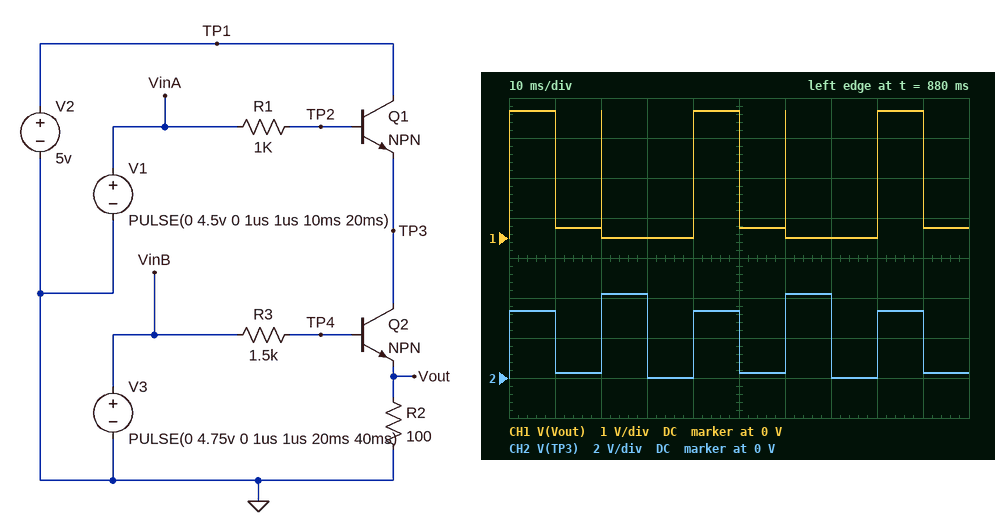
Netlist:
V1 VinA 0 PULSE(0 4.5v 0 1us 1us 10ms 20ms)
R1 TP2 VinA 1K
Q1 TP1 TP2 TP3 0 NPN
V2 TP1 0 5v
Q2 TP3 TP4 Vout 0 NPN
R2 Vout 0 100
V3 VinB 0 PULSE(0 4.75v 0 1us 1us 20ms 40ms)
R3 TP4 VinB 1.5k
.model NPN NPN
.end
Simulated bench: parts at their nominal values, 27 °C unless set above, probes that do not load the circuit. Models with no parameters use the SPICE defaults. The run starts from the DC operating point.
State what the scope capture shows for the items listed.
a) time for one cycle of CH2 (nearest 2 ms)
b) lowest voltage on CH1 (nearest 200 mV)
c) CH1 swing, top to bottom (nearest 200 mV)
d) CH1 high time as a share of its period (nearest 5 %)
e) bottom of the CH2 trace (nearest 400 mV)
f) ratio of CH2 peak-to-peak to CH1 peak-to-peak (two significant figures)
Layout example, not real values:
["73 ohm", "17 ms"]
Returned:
["20 ms", "0 V", "3.2 V", "25 %", "0 V", "1.3"]
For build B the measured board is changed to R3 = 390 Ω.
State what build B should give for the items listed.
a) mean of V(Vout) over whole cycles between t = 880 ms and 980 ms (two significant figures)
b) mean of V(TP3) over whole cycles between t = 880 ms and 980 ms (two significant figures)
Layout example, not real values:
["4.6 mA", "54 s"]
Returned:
["1.0 V", "2.1 V"]
